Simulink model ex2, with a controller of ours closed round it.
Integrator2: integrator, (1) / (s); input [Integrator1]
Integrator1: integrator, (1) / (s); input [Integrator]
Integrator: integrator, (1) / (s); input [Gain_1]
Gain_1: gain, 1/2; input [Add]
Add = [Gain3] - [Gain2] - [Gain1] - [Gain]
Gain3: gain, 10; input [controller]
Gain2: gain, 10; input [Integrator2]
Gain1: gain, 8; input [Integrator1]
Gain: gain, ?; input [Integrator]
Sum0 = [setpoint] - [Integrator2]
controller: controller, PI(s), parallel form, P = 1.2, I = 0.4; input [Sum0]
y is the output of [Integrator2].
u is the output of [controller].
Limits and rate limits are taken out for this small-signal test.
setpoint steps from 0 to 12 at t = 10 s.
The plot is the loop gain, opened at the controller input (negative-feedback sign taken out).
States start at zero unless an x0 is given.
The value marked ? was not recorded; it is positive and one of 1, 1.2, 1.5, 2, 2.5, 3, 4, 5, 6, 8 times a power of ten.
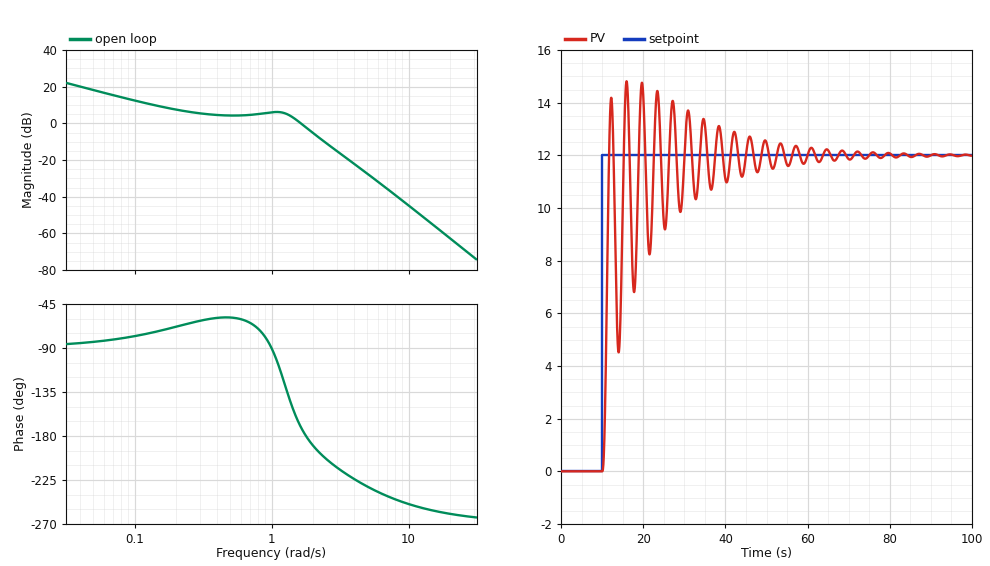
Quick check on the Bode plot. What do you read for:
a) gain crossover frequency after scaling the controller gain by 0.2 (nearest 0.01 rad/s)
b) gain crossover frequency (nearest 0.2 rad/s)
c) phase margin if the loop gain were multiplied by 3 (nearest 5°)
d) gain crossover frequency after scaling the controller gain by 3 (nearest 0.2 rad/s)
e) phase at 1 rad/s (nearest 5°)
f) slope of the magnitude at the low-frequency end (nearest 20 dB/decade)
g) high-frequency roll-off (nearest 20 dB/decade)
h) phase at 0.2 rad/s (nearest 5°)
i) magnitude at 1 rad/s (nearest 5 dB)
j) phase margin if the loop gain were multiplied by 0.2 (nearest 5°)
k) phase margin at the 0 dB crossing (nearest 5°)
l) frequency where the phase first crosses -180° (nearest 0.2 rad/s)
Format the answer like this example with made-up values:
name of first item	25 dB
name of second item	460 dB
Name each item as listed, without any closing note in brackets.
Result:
gain crossover frequency after scaling the controller gain by 0.2	0.08 rad/s
gain crossover frequency	1.6 rad/s
phase margin if the loop gain were multiplied by 3	-20°
gain crossover frequency after scaling the controller gain by 3	2.4 rad/s
phase at 1 rad/s	-90°
slope of the magnitude at the low-frequency end	-20 dB/decade
high-frequency roll-off	-60 dB/decade
phase at 0.2 rad/s	-70°
magnitude at 1 rad/s	5 dB
phase margin if the loop gain were multiplied by 0.2	100°
phase margin at the 0 dB crossing	10°
frequency where the phase first crosses -180°	1.8 rad/s
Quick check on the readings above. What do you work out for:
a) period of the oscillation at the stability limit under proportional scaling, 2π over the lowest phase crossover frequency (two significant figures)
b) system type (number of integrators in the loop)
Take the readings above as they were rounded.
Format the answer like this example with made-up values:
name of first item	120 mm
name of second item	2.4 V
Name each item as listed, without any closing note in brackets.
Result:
period of the oscillation at the stability limit under proportional scaling, 2π over the lowest phase crossover frequency	3.5 s
system type	1
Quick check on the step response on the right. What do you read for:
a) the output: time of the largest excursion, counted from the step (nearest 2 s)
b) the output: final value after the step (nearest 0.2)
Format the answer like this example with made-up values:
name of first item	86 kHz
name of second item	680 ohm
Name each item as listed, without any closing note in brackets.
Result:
the output: time of the largest excursion, counted from the step	6 s
the output: final value after the step	12.0
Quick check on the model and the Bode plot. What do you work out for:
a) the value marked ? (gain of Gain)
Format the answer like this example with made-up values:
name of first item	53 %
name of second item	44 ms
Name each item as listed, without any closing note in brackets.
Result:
the value marked ?	8
